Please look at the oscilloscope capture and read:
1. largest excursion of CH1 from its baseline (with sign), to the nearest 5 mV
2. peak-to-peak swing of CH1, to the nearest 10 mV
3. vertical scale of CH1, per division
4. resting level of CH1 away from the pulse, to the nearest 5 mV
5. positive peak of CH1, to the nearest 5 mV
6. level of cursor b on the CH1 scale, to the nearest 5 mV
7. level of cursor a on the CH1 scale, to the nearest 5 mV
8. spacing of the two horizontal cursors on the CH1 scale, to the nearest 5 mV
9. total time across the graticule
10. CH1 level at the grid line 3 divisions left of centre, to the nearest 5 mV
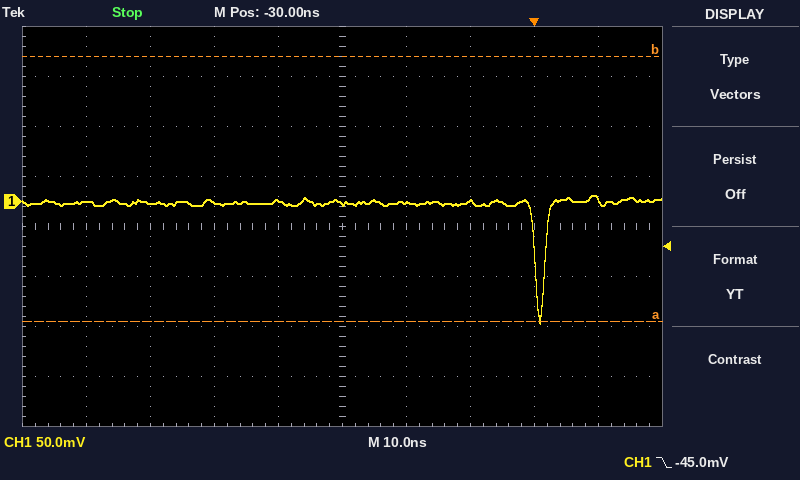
-120 mV
130 mV
50 mV
0 mV
5 mV
145 mV
-120 mV
265 mV
100 ns
0 mV
